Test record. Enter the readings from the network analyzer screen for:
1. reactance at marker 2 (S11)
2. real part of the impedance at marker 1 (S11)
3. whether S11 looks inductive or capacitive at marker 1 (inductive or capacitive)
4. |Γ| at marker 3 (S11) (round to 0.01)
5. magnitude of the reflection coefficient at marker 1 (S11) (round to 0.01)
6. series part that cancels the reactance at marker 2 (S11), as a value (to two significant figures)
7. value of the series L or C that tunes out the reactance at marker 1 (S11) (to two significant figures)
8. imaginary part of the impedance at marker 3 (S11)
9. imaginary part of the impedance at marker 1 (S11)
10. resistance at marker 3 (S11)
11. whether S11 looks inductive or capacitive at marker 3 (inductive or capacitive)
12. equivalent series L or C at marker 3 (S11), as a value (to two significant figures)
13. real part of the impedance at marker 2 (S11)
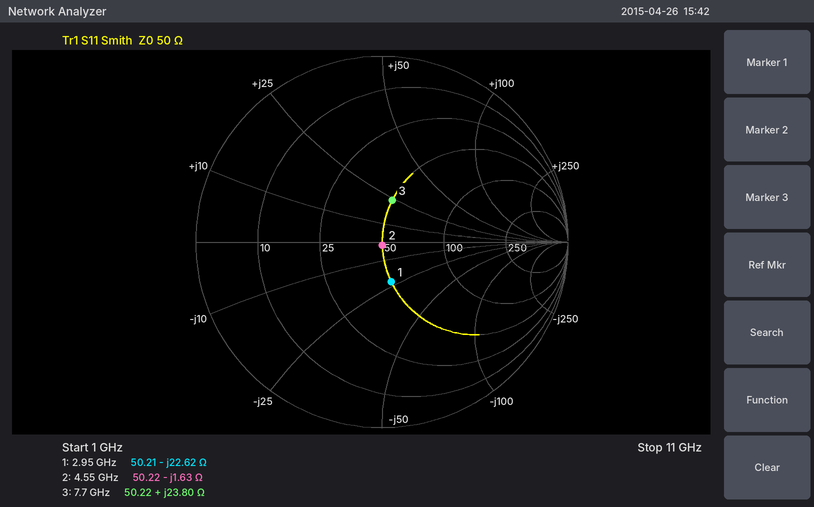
-1.63 Ω
50.21 Ω
capacitive
0.23
0.22
57 pH
1.2 nH
+23.80 Ω
-22.62 Ω
50.22 Ω
inductive
490 pH
50.22 Ω
